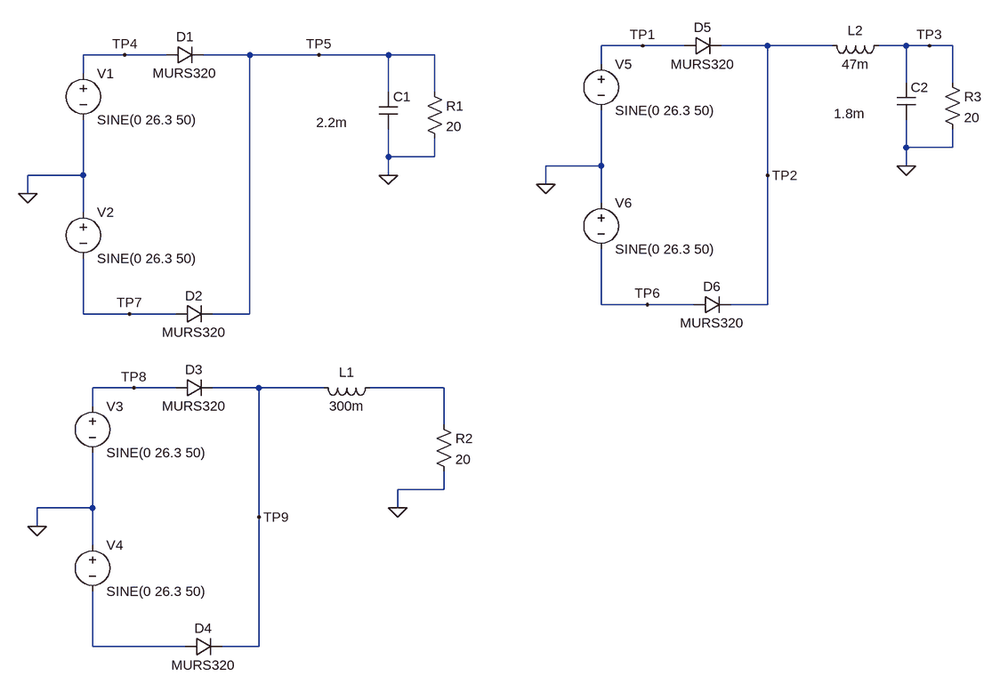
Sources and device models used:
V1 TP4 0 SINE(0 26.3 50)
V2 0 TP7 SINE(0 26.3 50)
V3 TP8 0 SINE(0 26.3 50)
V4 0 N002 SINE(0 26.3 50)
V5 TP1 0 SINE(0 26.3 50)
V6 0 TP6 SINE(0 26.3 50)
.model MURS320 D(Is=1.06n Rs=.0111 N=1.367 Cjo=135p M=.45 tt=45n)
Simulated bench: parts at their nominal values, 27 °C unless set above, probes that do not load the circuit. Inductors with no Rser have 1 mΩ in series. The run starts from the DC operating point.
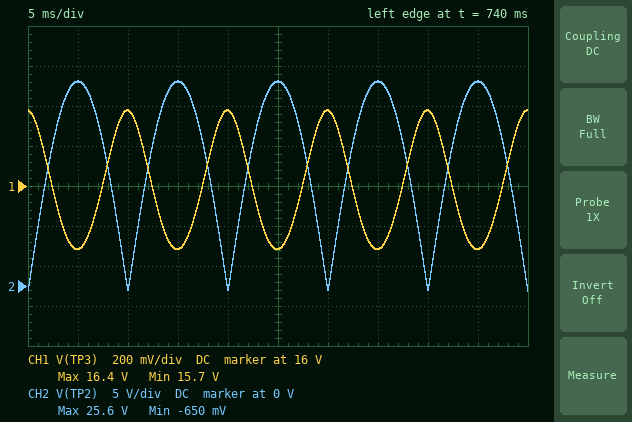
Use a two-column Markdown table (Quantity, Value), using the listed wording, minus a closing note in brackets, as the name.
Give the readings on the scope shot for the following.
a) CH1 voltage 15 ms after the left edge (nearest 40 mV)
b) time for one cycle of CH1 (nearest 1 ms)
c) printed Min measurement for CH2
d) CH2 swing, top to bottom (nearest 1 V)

| Quantity | Value |
|---|---|
| CH1 voltage 15 ms after the left edge | 15.68 V |
| time for one cycle of CH1 | 10 ms |
| printed Min measurement for CH2 | -650 mV |
| CH2 swing, top to bottom | 26 V |
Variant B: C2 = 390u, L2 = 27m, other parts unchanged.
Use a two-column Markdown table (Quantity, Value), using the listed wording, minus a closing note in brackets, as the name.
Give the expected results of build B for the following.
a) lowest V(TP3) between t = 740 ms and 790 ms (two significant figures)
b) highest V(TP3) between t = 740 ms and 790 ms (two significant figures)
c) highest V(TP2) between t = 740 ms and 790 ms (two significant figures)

| Quantity | Value |
|---|---|
| lowest V(TP3) between t = 740 ms and 790 ms | 13 V |
| highest V(TP3) between t = 740 ms and 790 ms | 20 V |
| highest V(TP2) between t = 740 ms and 790 ms | 26 V |
